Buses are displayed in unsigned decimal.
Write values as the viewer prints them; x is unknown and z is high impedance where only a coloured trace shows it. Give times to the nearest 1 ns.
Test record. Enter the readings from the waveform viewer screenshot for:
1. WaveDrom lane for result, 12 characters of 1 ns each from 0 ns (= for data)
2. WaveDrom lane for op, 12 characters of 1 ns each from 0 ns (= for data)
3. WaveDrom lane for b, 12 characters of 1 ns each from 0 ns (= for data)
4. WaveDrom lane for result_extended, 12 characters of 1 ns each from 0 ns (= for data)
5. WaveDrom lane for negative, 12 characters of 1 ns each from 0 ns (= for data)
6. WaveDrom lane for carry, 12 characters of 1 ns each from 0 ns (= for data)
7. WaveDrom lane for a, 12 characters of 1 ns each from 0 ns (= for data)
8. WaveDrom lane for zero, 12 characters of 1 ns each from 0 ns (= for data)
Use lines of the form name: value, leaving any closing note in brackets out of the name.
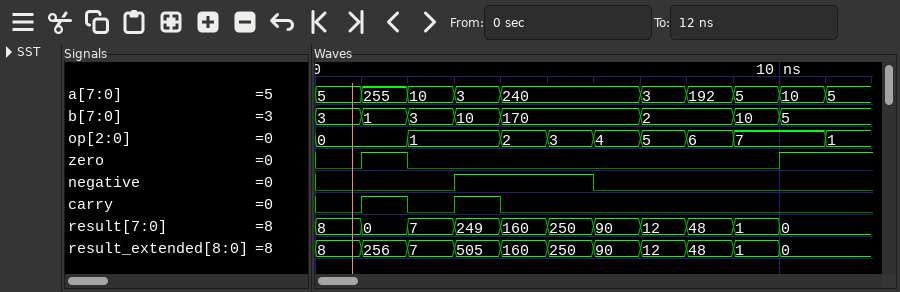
WaveDrom lane for result, 12 characters of 1 ns each from 0 ns: {name: 'result', wave: '===========.', data: '8 0 7 249 160 250 90 12 48 1 0'}
WaveDrom lane for op, 12 characters of 1 ns each from 0 ns: {name: 'op', wave: '=.=.======.=', data: '0 1 2 3 4 5 6 7 1'}
WaveDrom lane for b, 12 characters of 1 ns each from 0 ns: {name: 'b', wave: '=====..=.==.', data: '3 1 3 10 170 2 10 5'}
WaveDrom lane for result_extended, 12 characters of 1 ns each from 0 ns: {name: 'result_extended', wave: '===========.', data: '8 256 7 505 160 250 90 12 48 1 0'}
WaveDrom lane for negative, 12 characters of 1 ns each from 0 ns: {name: 'negative', wave: '0..1..0.....'}
WaveDrom lane for carry, 12 characters of 1 ns each from 0 ns: {name: 'carry', wave: '01010.......'}
WaveDrom lane for a, 12 characters of 1 ns each from 0 ns: {name: 'a', wave: '=====..=====', data: '5 255 10 3 240 3 192 5 10 5'}
WaveDrom lane for zero, 12 characters of 1 ns each from 0 ns: {name: 'zero', wave: '010.......1.'}
